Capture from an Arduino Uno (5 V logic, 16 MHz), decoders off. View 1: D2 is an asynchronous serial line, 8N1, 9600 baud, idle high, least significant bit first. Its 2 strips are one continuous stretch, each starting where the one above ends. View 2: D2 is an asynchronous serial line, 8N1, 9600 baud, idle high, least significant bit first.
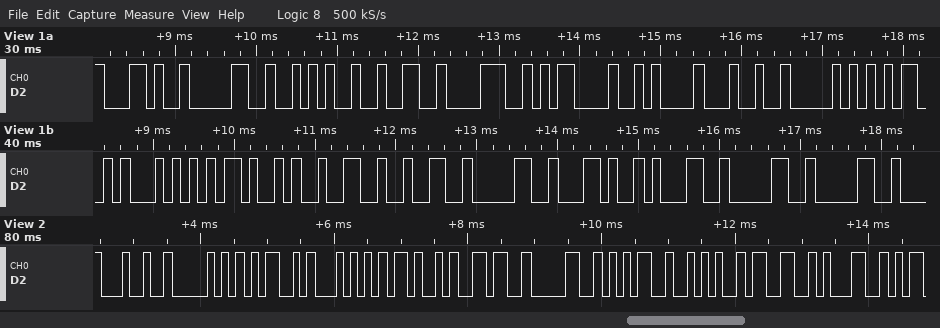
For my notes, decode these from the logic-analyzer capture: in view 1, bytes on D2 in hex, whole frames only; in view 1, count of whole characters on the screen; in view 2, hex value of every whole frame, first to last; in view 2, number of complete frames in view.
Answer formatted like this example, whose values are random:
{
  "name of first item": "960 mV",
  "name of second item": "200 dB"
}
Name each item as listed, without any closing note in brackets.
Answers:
{
  "in view 1, bytes on D2 in hex, whole frames only": "2C 30 2A 32 38 0D 0A 24 50 4D 54 4B 32 32 30 2C 31 30 30",
  "in view 1, count of whole characters on the screen": "19",
  "in view 2, hex value of every whole frame, first to last": "0x24 0x50 0x4D 0x54 0x4B 0x36 0x30 0x35 0x2A 0x33 0x31",
  "in view 2, number of complete frames in view": "11"
}
